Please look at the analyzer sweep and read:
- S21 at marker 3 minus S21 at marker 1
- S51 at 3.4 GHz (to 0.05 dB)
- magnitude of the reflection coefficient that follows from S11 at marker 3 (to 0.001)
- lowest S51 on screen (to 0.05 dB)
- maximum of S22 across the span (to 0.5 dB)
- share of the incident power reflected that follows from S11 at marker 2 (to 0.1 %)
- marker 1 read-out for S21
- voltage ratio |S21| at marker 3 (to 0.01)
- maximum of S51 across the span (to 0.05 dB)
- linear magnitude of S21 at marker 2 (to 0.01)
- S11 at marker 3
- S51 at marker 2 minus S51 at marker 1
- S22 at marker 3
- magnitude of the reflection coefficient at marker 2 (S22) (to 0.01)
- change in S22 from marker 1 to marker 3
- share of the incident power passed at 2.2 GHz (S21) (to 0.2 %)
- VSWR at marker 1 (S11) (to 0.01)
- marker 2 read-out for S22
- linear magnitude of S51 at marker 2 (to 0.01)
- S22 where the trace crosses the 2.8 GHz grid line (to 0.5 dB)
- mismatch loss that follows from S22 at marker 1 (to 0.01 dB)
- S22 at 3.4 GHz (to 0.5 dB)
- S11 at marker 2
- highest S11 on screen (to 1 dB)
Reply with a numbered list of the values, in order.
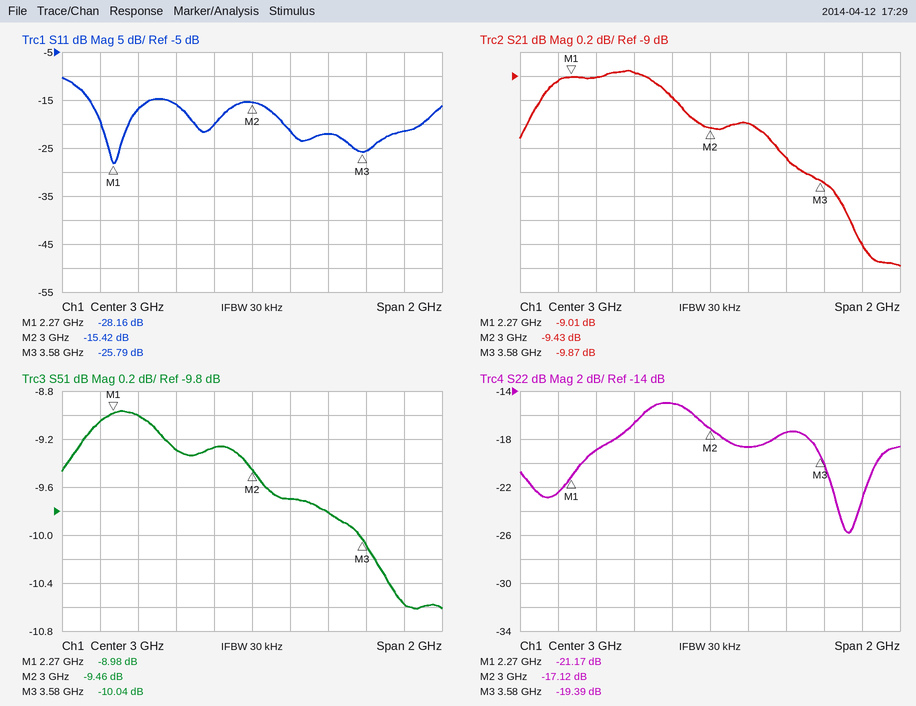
1. -0.86 dB
2. -9.80 dB
3. 0.051
4. -10.60 dB
5. -15.0 dB
6. 2.9 %
7. -9.01 dB
8. 0.32
9. -8.95 dB
10. 0.34
11. -25.79 dB
12. -0.48 dB
13. -19.39 dB
14. 0.14
15. 1.78 dB
16. 12.4 %
17. 1.08
18. -17.12 dB
19. 0.34
20. -15.0 dB
21. 0.03 dB
22. -17.5 dB
23. -15.42 dB
24. -10 dB
